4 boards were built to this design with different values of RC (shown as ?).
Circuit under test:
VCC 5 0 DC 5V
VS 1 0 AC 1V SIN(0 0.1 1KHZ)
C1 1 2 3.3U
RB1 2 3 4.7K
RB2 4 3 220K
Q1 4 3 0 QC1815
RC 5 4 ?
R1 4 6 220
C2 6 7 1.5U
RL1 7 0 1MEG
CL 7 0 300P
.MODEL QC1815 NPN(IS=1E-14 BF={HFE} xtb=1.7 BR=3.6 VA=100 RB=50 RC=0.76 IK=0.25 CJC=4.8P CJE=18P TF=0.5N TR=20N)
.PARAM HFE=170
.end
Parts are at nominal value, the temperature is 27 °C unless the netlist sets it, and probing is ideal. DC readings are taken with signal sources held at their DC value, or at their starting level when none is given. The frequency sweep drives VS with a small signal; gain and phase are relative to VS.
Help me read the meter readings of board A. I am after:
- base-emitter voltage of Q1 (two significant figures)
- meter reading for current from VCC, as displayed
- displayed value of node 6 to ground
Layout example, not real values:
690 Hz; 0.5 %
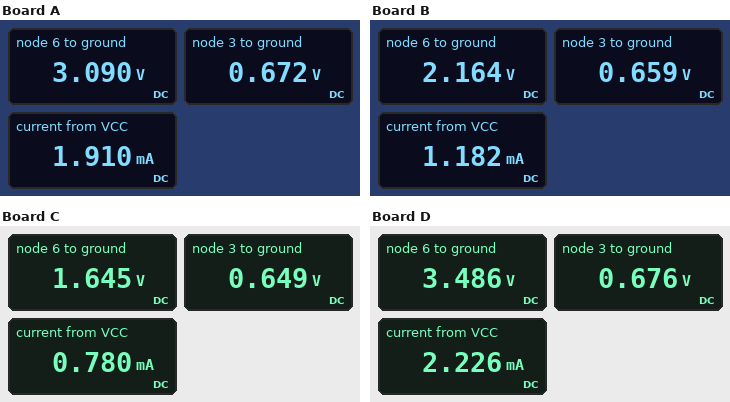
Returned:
670 mV; 1.910 mA; 3.090 V
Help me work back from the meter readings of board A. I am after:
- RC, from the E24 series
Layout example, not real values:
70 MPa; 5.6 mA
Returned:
1 kΩ
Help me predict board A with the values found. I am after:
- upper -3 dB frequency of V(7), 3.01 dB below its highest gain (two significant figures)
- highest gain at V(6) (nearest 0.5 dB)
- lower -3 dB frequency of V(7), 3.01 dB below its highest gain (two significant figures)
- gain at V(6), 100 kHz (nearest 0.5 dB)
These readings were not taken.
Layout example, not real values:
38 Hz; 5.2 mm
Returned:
330 kHz; 24.0 dB; 8.0 Hz; 23.5 dB
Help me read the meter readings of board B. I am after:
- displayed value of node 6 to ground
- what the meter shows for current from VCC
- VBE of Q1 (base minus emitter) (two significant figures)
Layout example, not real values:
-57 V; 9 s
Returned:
2.164 V; 1.182 mA; 660 mV
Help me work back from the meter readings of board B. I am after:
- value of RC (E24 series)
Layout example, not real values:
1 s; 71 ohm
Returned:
2.4 kΩ
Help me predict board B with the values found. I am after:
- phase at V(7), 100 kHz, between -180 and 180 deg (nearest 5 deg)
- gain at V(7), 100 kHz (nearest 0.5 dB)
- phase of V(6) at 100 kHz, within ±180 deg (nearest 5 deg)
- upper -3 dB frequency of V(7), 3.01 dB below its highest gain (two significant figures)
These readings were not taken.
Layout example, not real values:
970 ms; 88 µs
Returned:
150 deg; 26.5 dB; 150 deg; 210 kHz
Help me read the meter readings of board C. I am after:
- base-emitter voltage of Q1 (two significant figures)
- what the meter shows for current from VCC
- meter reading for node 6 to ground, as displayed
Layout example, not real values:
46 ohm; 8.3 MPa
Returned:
650 mV; 0.780 mA; 1.645 V
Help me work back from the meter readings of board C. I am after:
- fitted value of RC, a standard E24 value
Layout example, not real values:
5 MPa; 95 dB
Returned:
4.3 kΩ
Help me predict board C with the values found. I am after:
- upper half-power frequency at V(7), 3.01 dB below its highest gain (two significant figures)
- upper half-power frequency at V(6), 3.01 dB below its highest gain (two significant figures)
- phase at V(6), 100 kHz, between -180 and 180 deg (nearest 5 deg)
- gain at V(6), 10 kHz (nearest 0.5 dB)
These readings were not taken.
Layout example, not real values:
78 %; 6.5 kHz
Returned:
160 kHz; 160 kHz; 145 deg; 28.5 dB
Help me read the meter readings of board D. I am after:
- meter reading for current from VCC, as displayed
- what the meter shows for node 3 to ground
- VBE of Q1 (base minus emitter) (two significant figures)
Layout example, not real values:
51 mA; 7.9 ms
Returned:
2.226 mA; 0.676 V; 680 mV
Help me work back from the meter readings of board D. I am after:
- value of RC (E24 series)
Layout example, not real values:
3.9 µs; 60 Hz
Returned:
680 Ω
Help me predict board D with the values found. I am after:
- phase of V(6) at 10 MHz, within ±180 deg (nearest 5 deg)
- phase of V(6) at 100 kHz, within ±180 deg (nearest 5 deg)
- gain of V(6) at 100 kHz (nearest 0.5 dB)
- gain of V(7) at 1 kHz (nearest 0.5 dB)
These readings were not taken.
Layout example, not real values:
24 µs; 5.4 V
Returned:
10 deg; 165 deg; 21.5 dB; 22.0 dB
